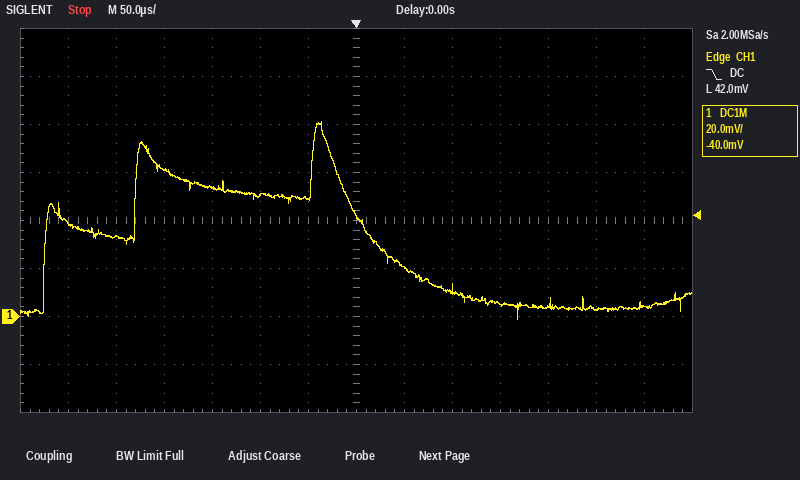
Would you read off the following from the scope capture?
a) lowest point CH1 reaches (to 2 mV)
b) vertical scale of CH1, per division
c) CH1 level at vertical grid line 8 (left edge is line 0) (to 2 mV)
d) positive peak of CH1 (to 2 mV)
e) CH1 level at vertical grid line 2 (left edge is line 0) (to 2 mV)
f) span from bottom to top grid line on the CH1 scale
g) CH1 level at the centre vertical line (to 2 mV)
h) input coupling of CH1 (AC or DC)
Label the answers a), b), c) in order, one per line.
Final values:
a) -2 mV
b) 20 mV
c) 20 mV
d) 82 mV
e) 34 mV
f) 160 mV
g) 42 mV
h) DC
